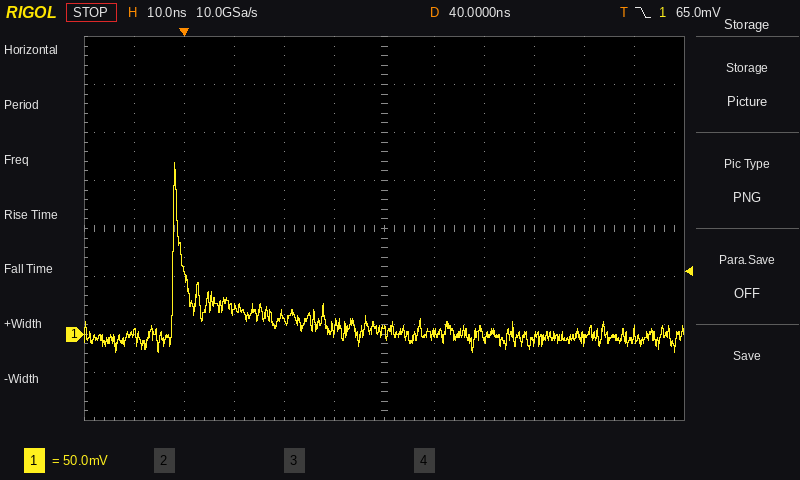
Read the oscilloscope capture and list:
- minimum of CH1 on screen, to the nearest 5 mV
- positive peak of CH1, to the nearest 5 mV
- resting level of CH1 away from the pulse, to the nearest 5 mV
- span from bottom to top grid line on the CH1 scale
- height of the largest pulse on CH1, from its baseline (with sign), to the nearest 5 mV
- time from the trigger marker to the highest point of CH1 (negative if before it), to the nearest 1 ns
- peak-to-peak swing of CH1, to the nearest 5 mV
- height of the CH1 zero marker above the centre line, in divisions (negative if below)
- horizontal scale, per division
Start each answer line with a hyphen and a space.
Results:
- -20 mV
- 180 mV
- 0 mV
- 400 mV
- +180 mV
- -2 ns
- 200 mV
- -2.2 div
- 10 ns
